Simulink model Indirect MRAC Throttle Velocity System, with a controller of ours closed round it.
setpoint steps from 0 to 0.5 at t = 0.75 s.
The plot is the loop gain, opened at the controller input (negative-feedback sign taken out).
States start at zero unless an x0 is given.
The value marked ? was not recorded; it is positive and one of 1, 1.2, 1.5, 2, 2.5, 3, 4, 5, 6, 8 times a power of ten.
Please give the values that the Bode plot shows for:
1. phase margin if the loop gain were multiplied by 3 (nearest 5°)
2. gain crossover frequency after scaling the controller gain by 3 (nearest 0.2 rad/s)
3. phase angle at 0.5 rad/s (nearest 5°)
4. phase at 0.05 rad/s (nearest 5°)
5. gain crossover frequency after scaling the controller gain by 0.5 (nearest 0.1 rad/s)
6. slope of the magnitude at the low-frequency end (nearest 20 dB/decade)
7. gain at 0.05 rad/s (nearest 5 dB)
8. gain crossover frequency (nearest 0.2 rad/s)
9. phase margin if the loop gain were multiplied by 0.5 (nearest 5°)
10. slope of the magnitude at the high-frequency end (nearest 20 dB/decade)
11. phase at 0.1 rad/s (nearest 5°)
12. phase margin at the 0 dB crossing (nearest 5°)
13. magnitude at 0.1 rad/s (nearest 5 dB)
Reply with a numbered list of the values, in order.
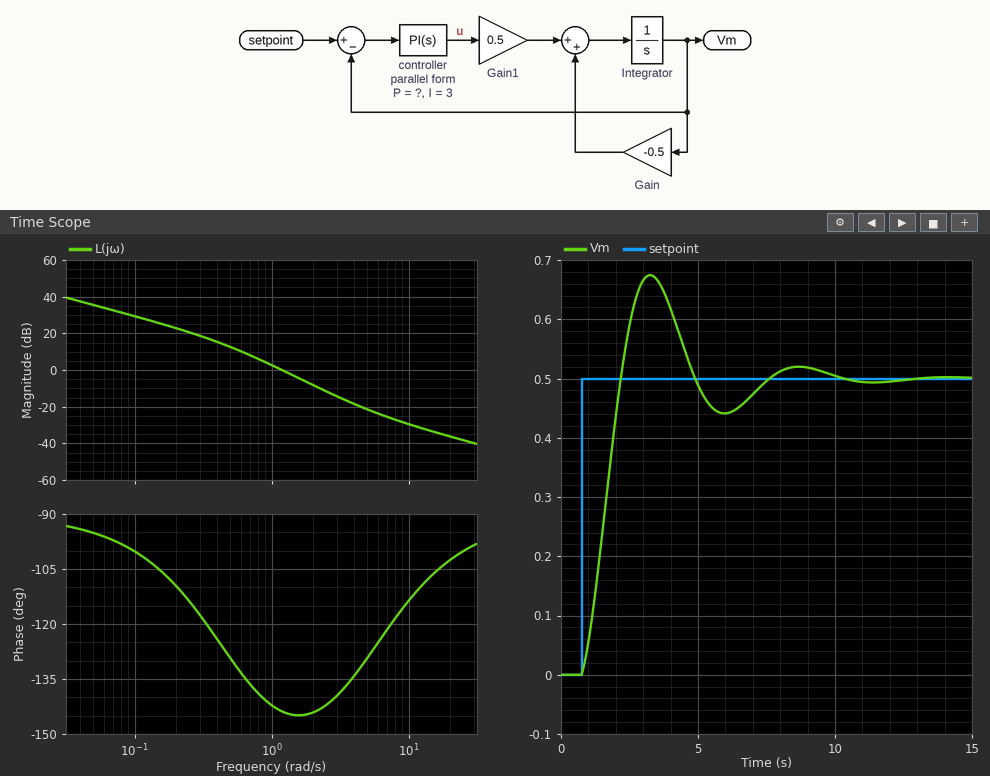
1. 35°
2. 2.2 rad/s
3. -130°
4. -95°
5. 0.8 rad/s
6. -20 dB/decade
7. 35 dB
8. 1.2 rad/s
9. 40°
10. -20 dB/decade
11. -100°
12. 35°
13. 30 dB
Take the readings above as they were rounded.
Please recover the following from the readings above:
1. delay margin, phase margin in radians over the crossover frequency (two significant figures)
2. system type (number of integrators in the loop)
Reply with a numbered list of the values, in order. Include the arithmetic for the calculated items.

1. 35 × π / 180 / 1.2 = 0.51 s
2. 1
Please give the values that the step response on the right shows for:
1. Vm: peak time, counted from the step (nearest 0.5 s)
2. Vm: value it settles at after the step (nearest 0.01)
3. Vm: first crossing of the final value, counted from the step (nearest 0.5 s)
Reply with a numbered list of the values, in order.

1. 2.5 s
2. 0.50
3. 1.5 s
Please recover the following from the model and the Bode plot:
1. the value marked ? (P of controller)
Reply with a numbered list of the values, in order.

1. 0.6
